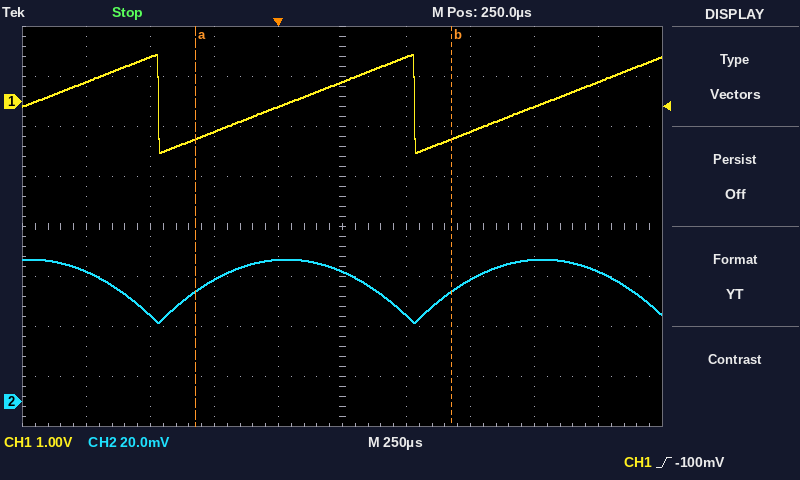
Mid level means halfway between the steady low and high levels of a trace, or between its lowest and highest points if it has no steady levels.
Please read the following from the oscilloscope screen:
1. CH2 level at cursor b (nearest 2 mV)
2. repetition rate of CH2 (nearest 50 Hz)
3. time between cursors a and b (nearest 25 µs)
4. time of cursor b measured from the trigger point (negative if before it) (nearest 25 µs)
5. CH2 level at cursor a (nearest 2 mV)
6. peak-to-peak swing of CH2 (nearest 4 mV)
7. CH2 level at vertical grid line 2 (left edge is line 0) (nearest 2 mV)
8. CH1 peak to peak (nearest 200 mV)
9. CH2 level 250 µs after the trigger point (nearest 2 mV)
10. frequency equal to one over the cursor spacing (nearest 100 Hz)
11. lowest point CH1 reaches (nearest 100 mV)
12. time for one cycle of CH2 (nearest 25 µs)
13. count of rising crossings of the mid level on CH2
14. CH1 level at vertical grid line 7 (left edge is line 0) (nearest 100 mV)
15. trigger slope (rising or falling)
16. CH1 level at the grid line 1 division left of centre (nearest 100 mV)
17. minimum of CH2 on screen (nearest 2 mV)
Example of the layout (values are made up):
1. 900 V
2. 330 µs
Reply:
1. 44 mV
2. 1.00 kHz
3. 1.000 ms
4. +675 µs
5. 44 mV
6. 24 mV
7. 34 mV
8. 2.0 V
9. 52 mV
10. 1.0 kHz
11. -1.0 V
12. 1.000 ms
13. 2
14. -600 mV
15. rising
16. -100 mV
17. 32 mV
